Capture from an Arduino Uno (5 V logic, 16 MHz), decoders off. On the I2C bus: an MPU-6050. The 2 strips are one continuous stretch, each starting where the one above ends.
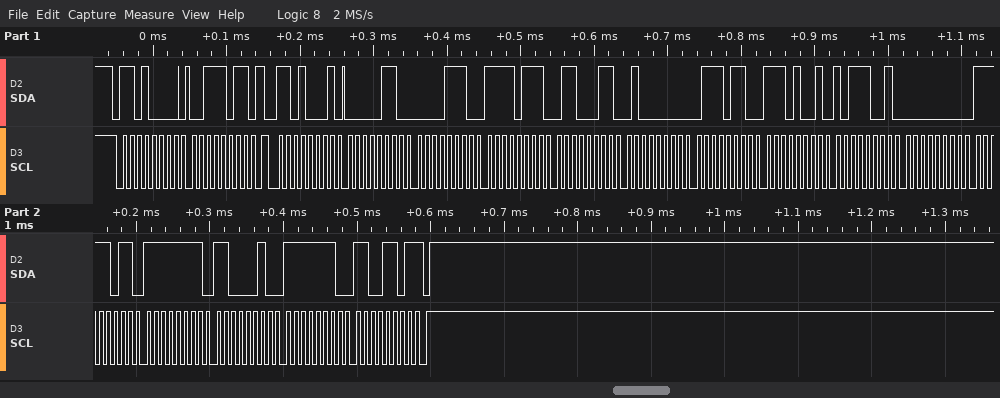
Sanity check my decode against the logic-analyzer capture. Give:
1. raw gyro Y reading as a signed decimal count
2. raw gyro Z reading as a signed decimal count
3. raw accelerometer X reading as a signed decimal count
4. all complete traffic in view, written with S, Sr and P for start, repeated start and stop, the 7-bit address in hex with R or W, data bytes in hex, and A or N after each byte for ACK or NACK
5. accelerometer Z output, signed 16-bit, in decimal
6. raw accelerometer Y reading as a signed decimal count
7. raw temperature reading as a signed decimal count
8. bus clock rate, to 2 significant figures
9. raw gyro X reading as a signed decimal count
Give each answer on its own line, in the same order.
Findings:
-62
-307
1550
S 68W A 3B A Sr 68R A 06 A 0E A F7 A 63 A 40 A 76 A E9 A B9 A 00 A FB A FF A C2 A FE A CD N P
16502
-2205
-5703
100 kHz
251
